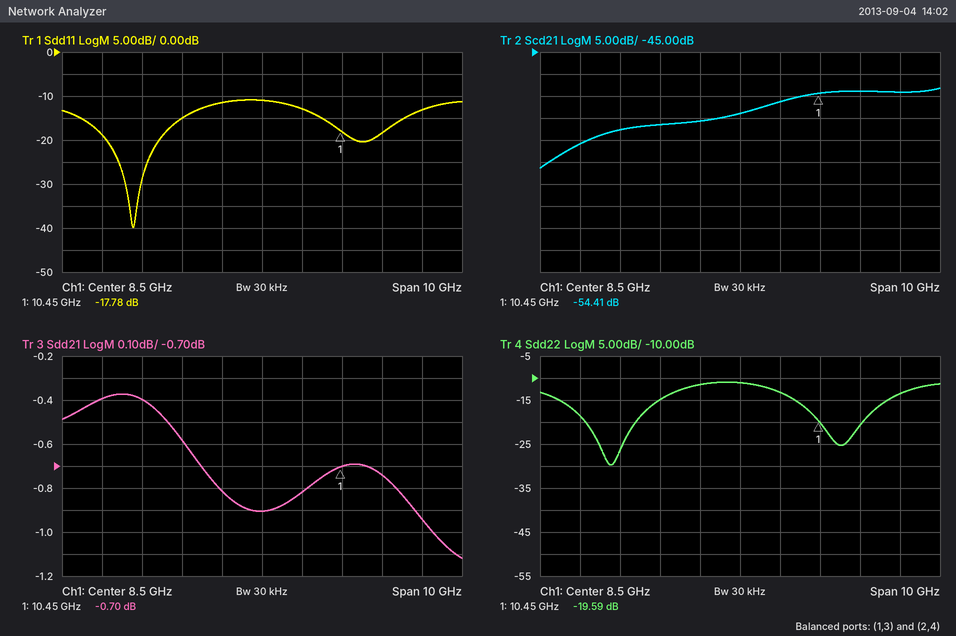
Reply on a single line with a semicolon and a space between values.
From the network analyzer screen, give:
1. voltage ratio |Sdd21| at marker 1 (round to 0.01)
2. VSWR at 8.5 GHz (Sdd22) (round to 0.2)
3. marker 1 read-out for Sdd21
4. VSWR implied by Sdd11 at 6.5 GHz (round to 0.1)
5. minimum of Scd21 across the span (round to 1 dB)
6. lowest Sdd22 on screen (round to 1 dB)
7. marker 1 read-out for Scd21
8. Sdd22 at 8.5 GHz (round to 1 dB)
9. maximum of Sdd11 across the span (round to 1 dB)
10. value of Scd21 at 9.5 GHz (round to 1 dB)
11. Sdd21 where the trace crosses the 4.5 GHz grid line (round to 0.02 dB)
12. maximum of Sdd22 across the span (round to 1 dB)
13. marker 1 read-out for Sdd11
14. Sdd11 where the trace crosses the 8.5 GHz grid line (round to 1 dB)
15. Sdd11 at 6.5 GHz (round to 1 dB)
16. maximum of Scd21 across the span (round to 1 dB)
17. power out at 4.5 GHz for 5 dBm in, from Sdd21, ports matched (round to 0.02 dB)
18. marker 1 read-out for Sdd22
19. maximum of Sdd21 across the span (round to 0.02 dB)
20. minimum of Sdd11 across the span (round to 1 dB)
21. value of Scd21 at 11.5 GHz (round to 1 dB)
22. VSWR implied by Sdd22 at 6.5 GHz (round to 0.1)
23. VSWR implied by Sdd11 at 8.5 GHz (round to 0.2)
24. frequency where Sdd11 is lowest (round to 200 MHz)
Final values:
0.92; 1.8; -0.70 dB; 1.4; -71 dB; -30 dB; -54.41 dB; -11 dB; -11 dB; -56 dB; -0.40 dB; -11 dB; -17.78 dB; -11 dB; -15 dB; -53 dB; 4.60 dBm; -19.59 dB; -0.38 dB; -40 dB; -54 dB; 1.4; 1.8; 5.2 GHz
